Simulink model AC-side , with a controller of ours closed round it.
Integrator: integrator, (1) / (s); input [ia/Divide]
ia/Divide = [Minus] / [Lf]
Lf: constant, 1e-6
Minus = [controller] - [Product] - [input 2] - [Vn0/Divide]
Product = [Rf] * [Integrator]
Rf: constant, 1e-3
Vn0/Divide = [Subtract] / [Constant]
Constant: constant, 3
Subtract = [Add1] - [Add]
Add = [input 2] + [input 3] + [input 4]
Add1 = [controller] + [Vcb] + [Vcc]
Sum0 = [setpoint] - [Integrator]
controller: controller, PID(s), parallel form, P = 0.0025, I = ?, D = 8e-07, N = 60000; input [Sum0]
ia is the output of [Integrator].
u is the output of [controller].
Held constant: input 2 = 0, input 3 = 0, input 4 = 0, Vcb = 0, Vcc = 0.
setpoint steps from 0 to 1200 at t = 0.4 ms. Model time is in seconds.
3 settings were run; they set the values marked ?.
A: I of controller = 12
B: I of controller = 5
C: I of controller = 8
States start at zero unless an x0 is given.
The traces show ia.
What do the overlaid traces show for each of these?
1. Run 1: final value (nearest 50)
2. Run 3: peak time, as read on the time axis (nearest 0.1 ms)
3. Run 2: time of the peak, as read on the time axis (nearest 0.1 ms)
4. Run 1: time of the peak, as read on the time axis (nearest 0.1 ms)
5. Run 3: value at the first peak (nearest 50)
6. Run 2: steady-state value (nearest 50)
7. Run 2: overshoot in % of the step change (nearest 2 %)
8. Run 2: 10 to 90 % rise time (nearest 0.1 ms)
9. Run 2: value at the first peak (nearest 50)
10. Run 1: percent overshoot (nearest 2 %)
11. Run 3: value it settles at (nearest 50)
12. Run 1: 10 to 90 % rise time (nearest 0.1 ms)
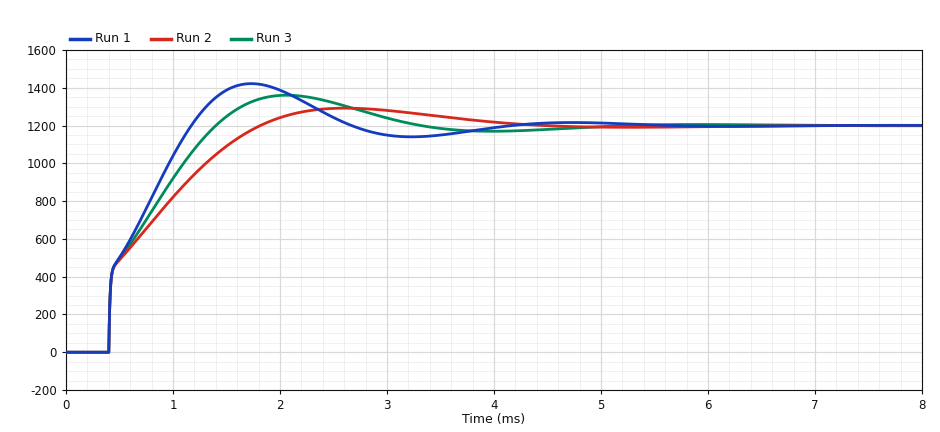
1200
2.1 ms
2.6 ms
1.7 ms
1350
1200
8 %
1.1 ms
1300
18 %
1200
0.6 ms
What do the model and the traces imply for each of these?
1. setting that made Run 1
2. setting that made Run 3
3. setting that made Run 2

A
C
B
